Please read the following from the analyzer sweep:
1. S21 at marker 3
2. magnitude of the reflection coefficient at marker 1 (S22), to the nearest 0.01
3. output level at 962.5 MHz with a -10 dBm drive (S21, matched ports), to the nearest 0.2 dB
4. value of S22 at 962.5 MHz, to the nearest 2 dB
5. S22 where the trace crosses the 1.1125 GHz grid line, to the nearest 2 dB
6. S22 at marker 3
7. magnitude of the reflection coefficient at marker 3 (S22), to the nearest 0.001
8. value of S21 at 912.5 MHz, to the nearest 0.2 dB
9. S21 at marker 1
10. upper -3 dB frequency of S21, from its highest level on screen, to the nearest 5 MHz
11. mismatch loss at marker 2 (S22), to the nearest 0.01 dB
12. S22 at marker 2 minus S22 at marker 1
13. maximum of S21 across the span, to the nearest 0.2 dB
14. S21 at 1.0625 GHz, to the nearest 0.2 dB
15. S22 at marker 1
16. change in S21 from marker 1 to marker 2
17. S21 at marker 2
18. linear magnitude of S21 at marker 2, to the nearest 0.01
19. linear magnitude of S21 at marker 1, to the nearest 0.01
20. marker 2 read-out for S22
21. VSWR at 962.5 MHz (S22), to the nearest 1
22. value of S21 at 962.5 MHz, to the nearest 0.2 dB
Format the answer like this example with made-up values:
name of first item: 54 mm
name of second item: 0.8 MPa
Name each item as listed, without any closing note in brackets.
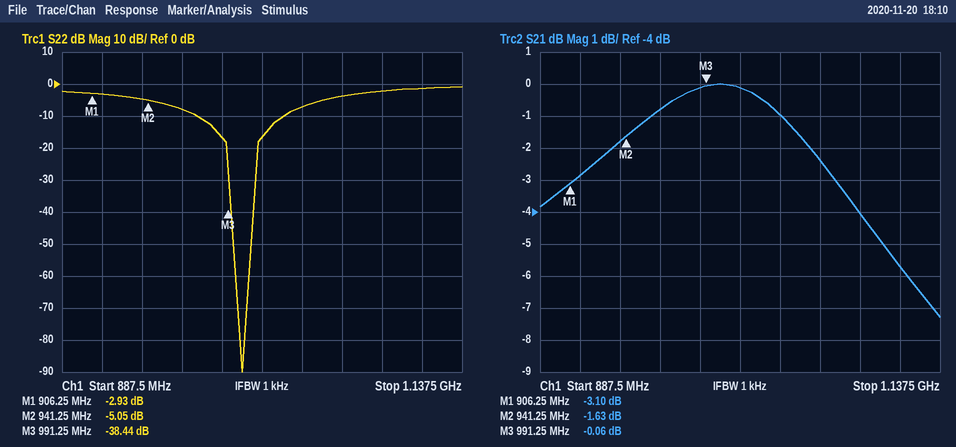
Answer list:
S21 at marker 3: -0.06 dB
magnitude of the reflection coefficient at marker 1 (S22), to the nearest 0.01: 0.71
output level at 962.5 MHz with a -10 dBm drive (S21, matched ports), to the nearest 0.2 dB: -10.8 dBm
value of S22 at 962.5 MHz, to the nearest 2 dB: -8 dB
S22 where the trace crosses the 1.1125 GHz grid line, to the nearest 2 dB: -2 dB
S22 at marker 3: -38.44 dB
magnitude of the reflection coefficient at marker 3 (S22), to the nearest 0.001: 0.012
value of S21 at 912.5 MHz, to the nearest 0.2 dB: -2.8 dB
S21 at marker 1: -3.10 dB
upper -3 dB frequency of S21, from its highest level on screen, to the nearest 5 MHz: 1.070 GHz
mismatch loss at marker 2 (S22), to the nearest 0.01 dB: 1.63 dB
S22 at marker 2 minus S22 at marker 1: -2.12 dB
maximum of S21 across the span, to the nearest 0.2 dB: 0.0 dB
S21 at 1.0625 GHz, to the nearest 0.2 dB: -2.4 dB
S22 at marker 1: -2.93 dB
change in S21 from marker 1 to marker 2: 1.47 dB
S21 at marker 2: -1.63 dB
linear magnitude of S21 at marker 2, to the nearest 0.01: 0.83
linear magnitude of S21 at marker 1, to the nearest 0.01: 0.70
marker 2 read-out for S22: -5.05 dB
VSWR at 962.5 MHz (S22), to the nearest 1: 2
value of S21 at 962.5 MHz, to the nearest 0.2 dB: -0.8 dB
